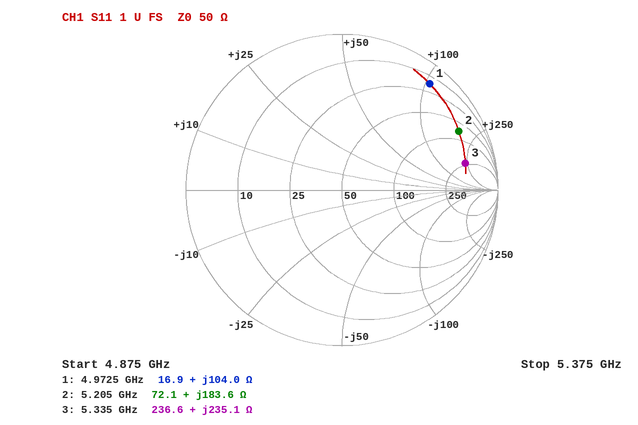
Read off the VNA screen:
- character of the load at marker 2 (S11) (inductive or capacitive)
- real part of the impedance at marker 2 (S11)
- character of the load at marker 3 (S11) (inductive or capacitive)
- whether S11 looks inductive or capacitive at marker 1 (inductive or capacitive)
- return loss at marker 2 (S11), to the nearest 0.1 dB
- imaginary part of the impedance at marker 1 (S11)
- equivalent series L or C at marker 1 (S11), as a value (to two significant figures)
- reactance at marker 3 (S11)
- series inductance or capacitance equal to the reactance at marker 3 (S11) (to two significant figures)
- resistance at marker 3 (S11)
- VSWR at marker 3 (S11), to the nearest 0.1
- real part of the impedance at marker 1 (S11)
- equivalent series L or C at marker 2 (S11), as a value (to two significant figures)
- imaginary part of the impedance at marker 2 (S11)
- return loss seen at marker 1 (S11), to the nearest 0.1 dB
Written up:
inductive
72.1 Ω
inductive
inductive
1.5 dB
+104.0 Ω
3.3 nH
+235.1 Ω
7.0 nH
236.6 Ω
9.5
16.9 Ω
5.6 nH
+183.6 Ω
1.1 dB
